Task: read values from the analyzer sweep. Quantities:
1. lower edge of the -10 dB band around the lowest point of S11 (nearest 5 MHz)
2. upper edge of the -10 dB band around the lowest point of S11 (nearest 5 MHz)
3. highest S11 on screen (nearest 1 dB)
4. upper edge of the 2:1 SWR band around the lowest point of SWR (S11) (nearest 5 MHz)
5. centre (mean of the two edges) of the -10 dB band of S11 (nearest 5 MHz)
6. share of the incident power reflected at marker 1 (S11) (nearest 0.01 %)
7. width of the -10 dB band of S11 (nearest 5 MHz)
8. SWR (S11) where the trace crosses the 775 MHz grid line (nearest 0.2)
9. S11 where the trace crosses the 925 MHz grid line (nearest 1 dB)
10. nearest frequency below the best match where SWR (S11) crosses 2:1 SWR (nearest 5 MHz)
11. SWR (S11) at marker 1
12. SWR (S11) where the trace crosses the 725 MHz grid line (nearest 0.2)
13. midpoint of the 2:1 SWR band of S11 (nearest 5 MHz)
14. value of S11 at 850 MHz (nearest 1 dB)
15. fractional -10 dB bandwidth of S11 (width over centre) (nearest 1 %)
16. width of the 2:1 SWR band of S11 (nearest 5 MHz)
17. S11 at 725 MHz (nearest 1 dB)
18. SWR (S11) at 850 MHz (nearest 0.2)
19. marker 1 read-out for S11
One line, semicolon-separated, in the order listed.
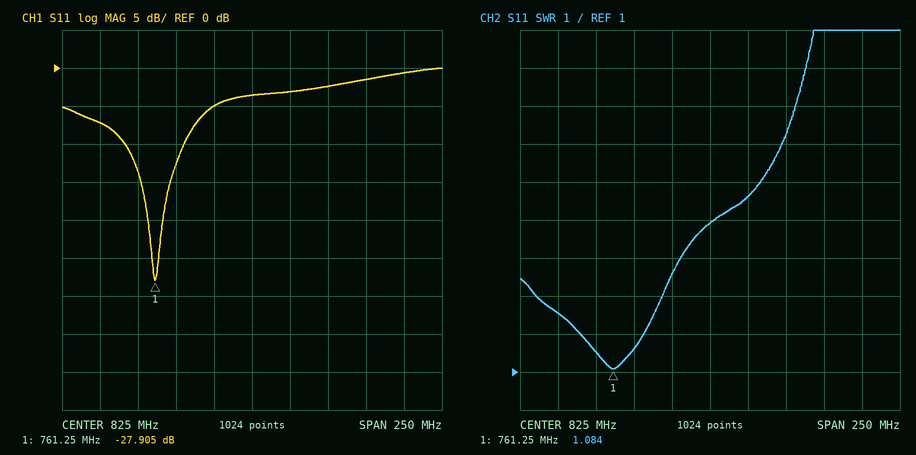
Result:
740 MHz; 780 MHz; 0 dB; 780 MHz; 760 MHz; 0.16 %; 40 MHz; 1.6; -1 dB; 740 MHz; 1.084; 2.6; 760 MHz; -3 dB; 5 %; 40 MHz; -7 dB; 5.6; -27.905 dB
